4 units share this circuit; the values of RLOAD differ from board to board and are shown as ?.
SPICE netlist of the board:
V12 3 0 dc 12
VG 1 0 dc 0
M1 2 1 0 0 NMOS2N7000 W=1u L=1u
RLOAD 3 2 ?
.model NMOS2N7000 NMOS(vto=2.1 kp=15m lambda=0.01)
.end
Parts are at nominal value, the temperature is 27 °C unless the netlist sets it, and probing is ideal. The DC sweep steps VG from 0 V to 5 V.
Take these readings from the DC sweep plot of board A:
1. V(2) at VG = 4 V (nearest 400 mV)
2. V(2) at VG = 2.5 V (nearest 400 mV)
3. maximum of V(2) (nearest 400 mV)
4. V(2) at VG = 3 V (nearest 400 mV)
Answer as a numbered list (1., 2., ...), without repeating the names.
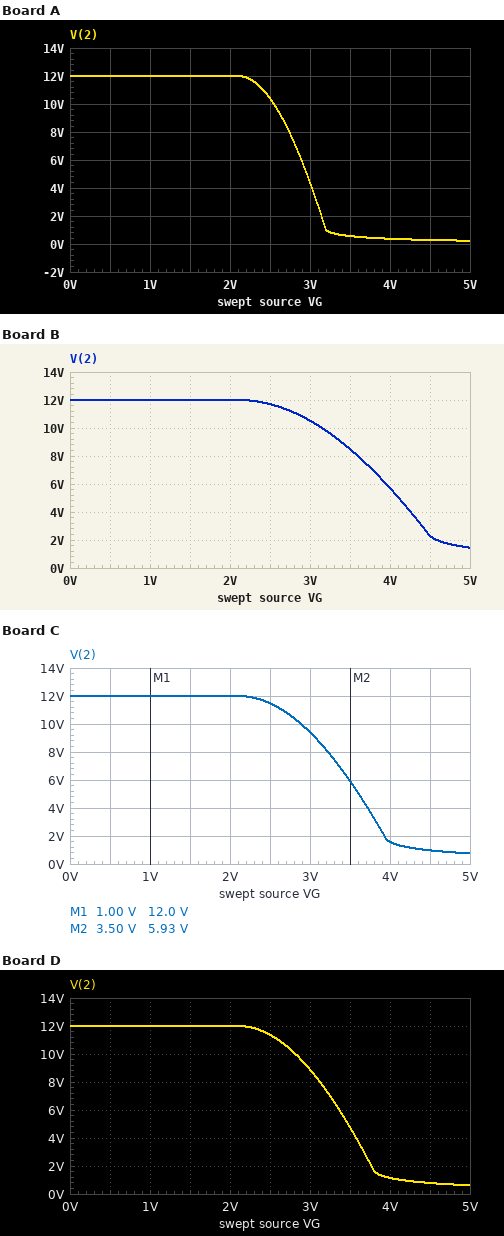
1. 400 mV
2. 10.4 V
3. 12.0 V
4. 4.4 V
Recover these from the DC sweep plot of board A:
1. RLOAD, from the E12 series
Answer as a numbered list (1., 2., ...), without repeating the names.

1. 1.2 kΩ
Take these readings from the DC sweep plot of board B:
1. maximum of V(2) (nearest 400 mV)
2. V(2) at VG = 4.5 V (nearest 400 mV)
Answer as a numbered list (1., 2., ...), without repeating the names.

1. 12.0 V
2. 2.4 V
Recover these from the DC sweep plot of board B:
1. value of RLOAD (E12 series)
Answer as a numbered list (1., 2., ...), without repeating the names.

1. 220 Ω
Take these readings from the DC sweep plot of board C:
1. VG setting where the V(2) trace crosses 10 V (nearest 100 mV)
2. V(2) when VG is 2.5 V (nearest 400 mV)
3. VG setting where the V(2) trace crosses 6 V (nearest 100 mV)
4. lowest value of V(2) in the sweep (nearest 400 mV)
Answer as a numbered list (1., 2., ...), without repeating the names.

1. 2.9 V
2. 11.6 V
3. 3.5 V
4. 800 mV
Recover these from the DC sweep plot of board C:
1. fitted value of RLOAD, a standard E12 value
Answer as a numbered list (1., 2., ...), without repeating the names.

1. 390 Ω
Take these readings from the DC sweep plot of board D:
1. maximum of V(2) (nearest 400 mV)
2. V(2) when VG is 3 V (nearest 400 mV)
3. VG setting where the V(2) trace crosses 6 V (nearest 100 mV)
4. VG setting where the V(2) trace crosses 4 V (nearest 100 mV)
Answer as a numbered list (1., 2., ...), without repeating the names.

1. 12.0 V
2. 8.8 V
3. 3.4 V
4. 3.6 V
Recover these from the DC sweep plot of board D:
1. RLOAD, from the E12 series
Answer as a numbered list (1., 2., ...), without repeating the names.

1. 470 Ω
